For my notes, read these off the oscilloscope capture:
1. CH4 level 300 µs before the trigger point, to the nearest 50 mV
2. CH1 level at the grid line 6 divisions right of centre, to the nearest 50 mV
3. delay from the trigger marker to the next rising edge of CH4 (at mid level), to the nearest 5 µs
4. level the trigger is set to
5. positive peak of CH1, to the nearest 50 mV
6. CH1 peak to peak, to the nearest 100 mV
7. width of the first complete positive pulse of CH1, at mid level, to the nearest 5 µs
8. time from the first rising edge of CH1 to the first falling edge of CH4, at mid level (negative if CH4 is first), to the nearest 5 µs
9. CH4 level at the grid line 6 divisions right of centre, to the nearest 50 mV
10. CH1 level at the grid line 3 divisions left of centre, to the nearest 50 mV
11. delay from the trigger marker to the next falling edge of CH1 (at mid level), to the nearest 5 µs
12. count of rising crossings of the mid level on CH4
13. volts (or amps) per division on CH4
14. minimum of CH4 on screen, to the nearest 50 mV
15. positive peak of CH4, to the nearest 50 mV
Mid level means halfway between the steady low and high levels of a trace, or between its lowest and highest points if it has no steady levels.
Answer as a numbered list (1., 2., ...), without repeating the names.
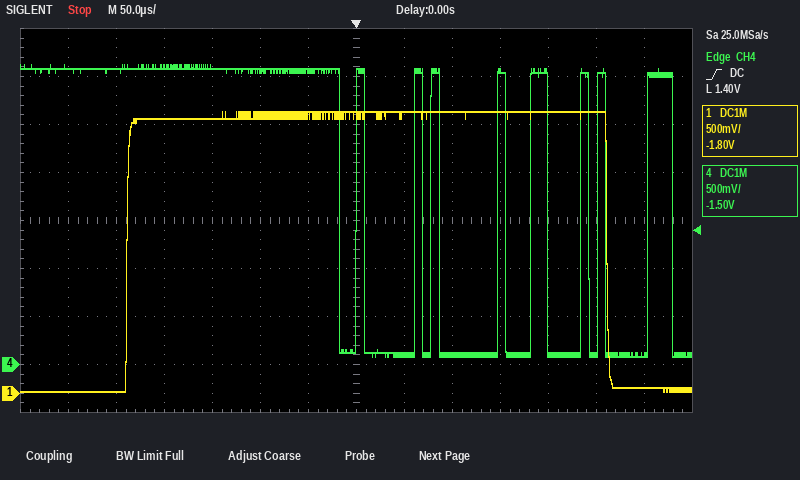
1. 3.10 V
2. 50 mV
3. 60 µs
4. 1.40 V
5. 2.95 V
6. 2.90 V
7. 500 µs
8. +220 µs
9. 100 mV
10. 2.85 V
11. 260 µs
12. 8
13. 500 mV
14. 100 mV
15. 3.10 V
